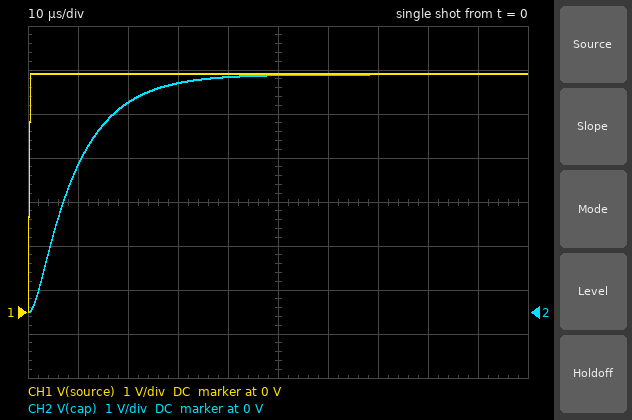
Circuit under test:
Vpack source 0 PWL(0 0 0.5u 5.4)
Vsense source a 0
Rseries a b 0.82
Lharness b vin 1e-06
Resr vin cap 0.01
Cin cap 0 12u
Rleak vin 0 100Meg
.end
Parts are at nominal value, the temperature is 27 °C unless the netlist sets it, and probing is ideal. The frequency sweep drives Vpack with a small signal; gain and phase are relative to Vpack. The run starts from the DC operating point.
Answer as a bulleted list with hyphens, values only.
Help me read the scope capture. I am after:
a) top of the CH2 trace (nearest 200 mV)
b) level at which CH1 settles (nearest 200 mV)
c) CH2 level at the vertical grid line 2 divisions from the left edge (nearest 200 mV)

- 5.4 V
- 5.4 V
- 4.8 V
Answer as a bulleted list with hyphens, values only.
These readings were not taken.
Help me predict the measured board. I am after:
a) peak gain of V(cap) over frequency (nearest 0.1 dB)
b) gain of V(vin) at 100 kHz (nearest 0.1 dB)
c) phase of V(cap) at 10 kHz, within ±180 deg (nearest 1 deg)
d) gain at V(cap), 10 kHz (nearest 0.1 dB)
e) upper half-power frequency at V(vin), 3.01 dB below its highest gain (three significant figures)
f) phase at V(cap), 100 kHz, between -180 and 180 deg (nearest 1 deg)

- 0 dB
- -17.2 dB
- -33 deg
- -1.1 dB
- 18.1 kHz
- -121 deg
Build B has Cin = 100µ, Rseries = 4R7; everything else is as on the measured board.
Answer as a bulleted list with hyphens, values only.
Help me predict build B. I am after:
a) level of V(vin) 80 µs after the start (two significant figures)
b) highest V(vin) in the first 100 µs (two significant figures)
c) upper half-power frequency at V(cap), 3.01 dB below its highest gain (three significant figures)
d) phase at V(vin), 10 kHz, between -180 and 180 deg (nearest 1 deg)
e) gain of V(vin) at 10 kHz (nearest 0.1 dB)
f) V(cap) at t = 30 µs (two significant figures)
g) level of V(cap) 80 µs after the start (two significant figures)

- 850 mV
- 1.0 V
- 338 Hz
- -85 deg
- -29.4 dB
- 330 mV
- 840 mV
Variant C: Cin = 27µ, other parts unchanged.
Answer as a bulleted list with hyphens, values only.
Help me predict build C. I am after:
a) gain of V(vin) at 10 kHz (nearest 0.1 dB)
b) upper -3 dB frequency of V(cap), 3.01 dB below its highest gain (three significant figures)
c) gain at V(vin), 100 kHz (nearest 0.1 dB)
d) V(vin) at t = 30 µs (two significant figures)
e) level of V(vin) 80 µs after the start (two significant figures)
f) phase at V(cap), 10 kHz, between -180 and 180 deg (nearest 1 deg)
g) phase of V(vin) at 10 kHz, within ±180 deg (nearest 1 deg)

- -4.4 dB
- 7.50 kHz
- -24.5 dB
- 4.0 V
- 5.3 V
- -58 deg
- -57 deg
